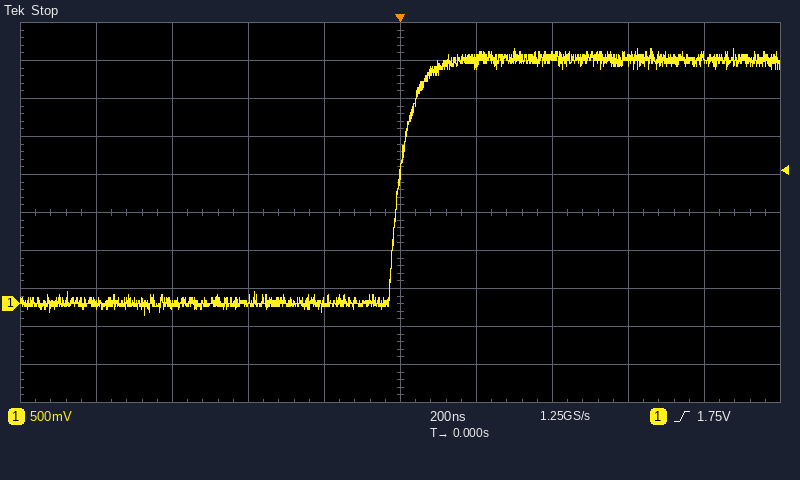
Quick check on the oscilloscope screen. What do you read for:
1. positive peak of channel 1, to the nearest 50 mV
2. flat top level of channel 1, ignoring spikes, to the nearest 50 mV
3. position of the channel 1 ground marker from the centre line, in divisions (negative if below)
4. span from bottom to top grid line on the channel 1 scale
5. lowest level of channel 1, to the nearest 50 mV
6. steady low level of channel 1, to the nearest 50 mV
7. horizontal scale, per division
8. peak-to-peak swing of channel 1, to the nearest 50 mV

3.35 V
3.20 V
-2.4 div
5 V
-150 mV
0 mV
200 ns
3.50 V
